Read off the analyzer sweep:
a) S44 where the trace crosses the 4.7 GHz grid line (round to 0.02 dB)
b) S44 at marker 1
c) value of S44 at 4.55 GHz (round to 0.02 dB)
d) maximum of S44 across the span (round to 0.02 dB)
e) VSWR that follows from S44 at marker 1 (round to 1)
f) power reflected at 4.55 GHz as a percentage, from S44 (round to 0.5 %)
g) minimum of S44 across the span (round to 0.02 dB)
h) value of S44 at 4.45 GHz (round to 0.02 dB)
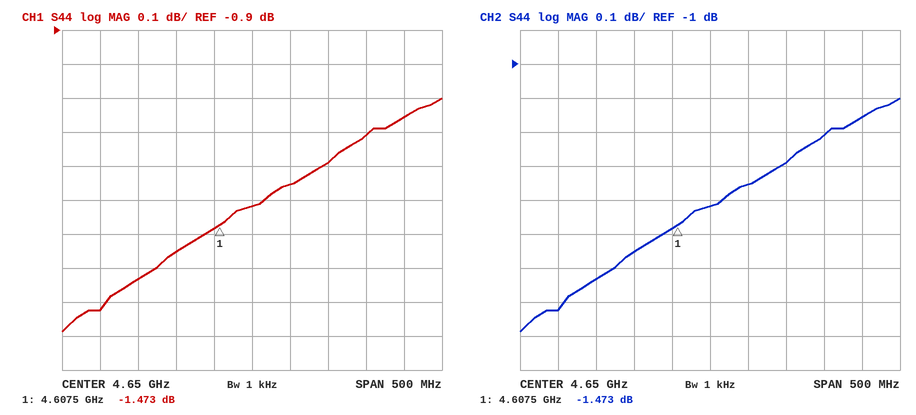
-1.36 dB
-1.473 dB
-1.56 dB
-1.10 dB
12
70.0 %
-1.78 dB
-1.72 dB
